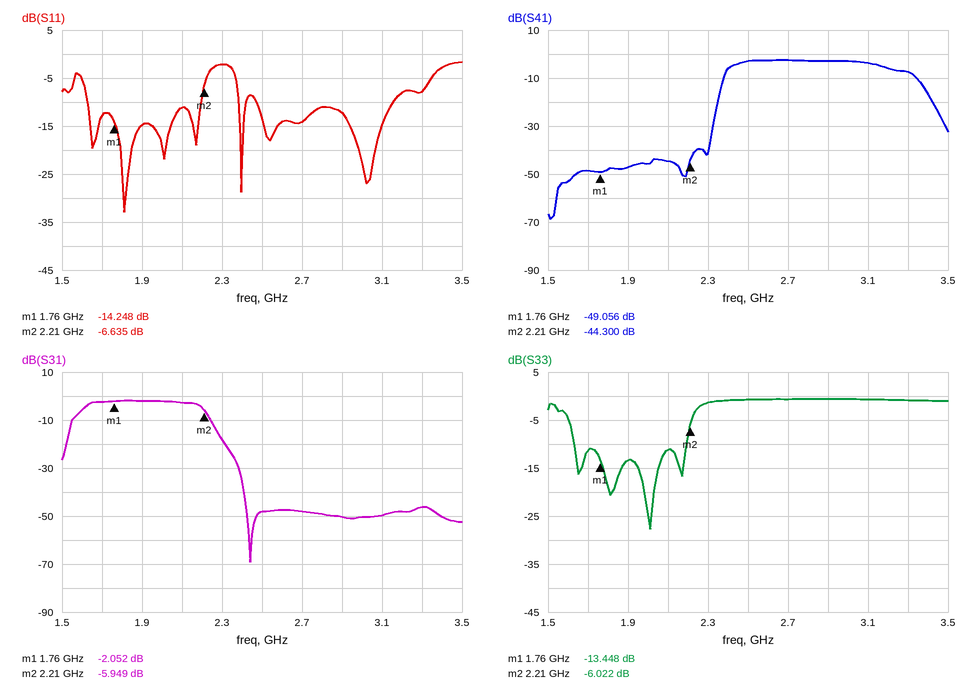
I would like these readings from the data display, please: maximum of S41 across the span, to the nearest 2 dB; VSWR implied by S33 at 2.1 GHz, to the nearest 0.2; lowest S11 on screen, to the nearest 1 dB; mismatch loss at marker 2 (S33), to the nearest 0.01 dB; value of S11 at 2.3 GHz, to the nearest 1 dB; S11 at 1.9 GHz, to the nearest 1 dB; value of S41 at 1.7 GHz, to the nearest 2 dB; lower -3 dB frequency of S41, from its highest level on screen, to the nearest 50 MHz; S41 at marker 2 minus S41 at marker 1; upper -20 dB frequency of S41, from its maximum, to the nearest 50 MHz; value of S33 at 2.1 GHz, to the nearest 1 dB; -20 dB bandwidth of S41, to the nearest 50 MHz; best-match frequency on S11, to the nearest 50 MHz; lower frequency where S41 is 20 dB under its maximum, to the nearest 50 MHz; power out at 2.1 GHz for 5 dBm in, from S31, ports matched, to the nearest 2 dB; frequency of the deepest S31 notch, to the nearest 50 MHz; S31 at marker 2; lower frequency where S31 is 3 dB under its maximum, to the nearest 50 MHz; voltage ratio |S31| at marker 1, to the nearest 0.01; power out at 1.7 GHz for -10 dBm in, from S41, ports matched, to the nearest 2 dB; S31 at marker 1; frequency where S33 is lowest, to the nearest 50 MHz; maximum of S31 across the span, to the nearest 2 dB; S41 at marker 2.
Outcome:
-2 dB
1.8
-33 dB
1.25 dB
-2 dB
-15 dB
-48 dB
2.40 GHz
4.756 dB
3.45 GHz
-11 dB
1.10 GHz
1.80 GHz
2.35 GHz
2 dBm
2.45 GHz
-5.949 dB
1.60 GHz
0.79
-58 dBm
-2.052 dB
2.00 GHz
-2 dB
-44.300 dB
